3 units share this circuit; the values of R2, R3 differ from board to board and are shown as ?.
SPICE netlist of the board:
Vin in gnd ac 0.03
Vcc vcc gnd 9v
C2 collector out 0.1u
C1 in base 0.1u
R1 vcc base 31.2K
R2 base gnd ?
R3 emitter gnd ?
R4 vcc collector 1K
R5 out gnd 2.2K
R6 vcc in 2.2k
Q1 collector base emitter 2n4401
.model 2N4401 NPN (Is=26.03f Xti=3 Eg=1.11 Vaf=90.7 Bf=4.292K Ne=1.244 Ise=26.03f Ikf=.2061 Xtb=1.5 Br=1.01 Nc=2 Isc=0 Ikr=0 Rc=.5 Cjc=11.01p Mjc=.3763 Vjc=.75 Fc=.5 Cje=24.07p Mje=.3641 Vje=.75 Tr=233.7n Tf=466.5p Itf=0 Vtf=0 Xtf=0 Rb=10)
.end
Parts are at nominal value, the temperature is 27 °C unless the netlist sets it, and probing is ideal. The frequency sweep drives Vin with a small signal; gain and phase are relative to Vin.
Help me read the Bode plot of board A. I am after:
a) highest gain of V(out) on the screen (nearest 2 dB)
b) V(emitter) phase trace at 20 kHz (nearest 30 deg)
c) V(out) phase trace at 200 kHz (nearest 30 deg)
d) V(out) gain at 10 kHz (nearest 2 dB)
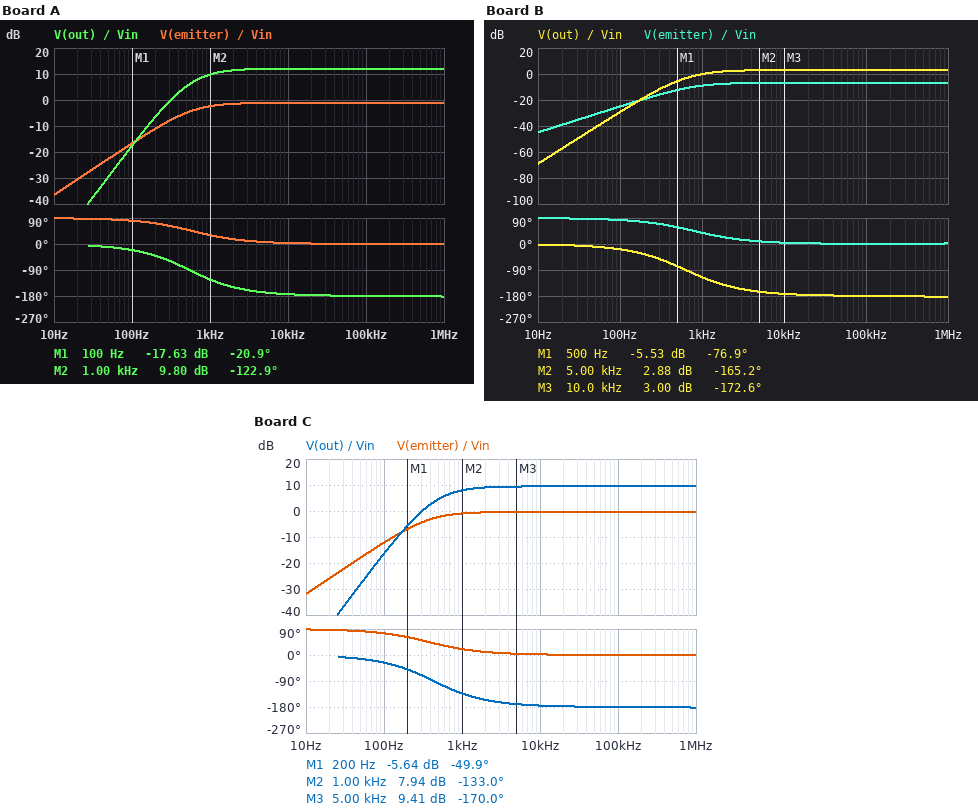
12 dB
0 deg
-180 deg
12 dB
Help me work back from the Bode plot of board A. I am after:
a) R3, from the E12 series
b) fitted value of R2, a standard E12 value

150 Ω
3.3 kΩ
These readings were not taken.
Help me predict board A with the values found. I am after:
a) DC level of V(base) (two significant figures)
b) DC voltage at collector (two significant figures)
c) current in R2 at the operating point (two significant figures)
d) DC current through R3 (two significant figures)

830 mV
7.7 V
250 µA
1.3 mA
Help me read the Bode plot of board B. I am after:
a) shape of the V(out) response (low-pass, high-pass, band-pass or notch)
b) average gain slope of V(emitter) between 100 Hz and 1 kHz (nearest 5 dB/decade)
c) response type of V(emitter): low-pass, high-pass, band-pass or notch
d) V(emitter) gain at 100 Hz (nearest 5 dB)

high-pass
15 dB/decade
high-pass
-25 dB
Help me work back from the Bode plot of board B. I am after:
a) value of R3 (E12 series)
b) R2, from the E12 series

220 Ω
2.2 kΩ
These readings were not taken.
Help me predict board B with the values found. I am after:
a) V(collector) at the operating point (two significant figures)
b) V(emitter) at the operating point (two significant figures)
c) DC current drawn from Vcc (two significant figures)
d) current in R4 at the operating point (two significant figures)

8.9 V
22 mV
4.5 mA
99 µA
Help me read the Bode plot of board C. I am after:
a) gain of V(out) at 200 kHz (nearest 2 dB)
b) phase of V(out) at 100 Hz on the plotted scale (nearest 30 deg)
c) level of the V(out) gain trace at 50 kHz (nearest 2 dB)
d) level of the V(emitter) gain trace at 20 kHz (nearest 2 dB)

10 dB
-30 deg
10 dB
0 dB
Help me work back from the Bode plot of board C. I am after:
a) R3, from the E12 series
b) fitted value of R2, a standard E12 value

220 Ω
5.6 kΩ
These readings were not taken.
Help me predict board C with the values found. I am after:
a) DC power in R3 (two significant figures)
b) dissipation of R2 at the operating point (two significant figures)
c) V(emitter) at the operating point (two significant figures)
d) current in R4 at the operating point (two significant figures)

1.8 mW
290 µW
620 mV
2.8 mA
